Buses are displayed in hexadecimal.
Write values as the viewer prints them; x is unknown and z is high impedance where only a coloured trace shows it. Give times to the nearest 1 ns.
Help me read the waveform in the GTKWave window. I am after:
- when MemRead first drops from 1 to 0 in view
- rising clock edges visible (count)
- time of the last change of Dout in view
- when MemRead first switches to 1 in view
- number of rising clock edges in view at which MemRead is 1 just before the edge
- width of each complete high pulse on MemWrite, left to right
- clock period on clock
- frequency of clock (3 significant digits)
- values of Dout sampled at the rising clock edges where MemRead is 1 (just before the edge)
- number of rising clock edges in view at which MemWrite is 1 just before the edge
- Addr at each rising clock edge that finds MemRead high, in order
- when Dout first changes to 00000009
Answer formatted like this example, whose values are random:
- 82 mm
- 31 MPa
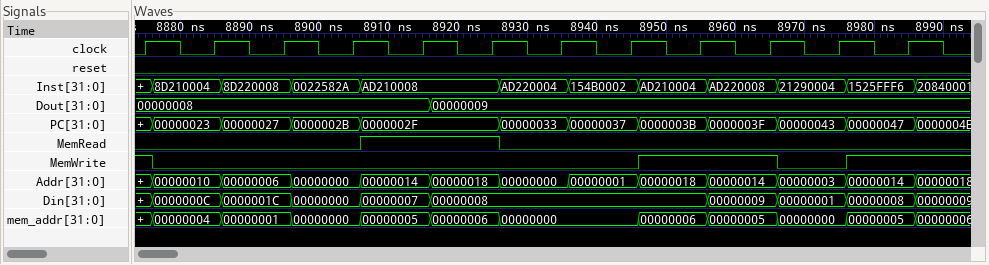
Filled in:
- 8926 ns
- 12
- 8916 ns
- 8906 ns
- 2
- 20 ns
- 10 ns
- 100 MHz
- 00000008, 00000009
- 4
- 00000014, 00000018
- 8916 ns
